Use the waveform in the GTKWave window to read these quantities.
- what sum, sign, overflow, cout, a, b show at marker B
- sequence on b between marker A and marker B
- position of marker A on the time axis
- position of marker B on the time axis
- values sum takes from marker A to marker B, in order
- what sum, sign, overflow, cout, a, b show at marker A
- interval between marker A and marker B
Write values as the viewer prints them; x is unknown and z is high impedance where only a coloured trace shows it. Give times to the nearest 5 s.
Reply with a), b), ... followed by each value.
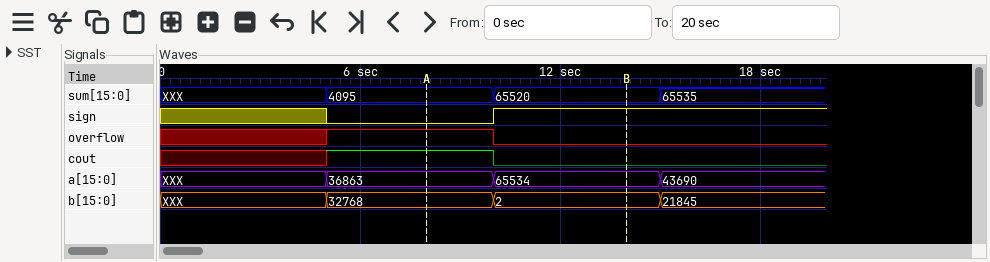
a) sum=65520, sign=1, overflow=0, cout=0, a=65534, b=2
b) 32768, 2
c) 10 s
d) 15 s
e) 4095, 65520
f) sum=4095, sign=0, overflow=1, cout=1, a=36863, b=32768
g) 5 s
